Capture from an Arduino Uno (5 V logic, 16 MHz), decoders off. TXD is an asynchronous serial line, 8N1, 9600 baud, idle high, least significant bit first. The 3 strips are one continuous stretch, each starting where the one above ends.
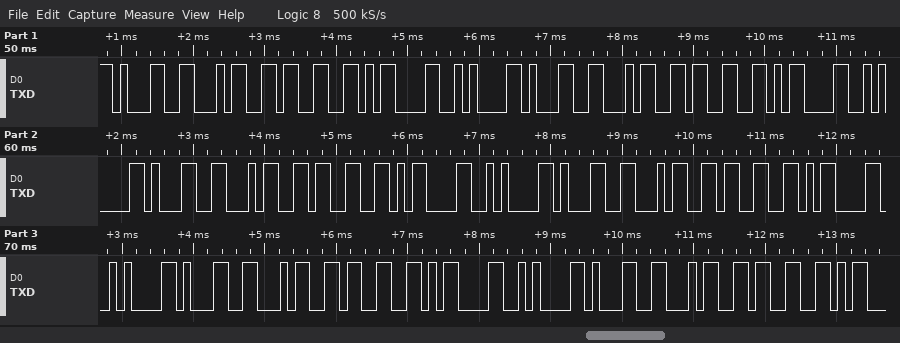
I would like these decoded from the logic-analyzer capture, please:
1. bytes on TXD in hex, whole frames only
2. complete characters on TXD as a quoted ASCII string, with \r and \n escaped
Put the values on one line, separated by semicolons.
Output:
0x31 0x34 0x33 0x0D 0x0A 0x31 0x34 0x33 0x0D 0x0A 0x31 0x34 0x33 0x0D 0x0A 0x31 0x34 0x33 0x0D 0x0A 0x31 0x34 0x33 0x0D 0x0A 0x31 0x34 0x33; "143\r\n143\r\n143\r\n143\r\n143\r\n143"
